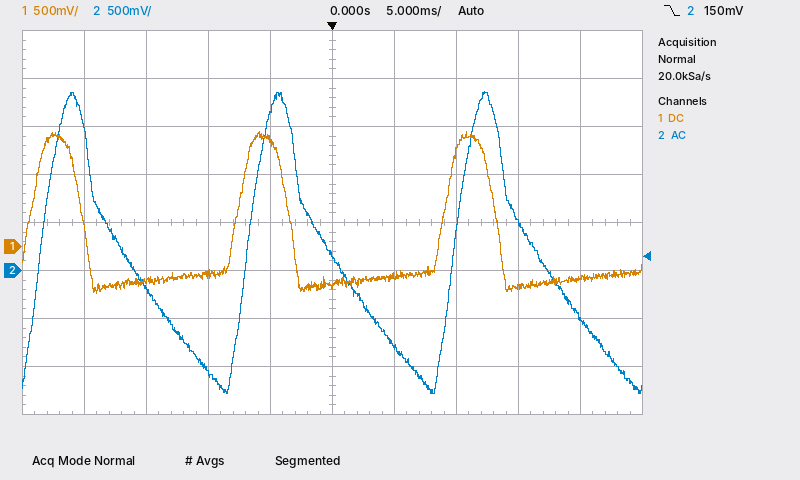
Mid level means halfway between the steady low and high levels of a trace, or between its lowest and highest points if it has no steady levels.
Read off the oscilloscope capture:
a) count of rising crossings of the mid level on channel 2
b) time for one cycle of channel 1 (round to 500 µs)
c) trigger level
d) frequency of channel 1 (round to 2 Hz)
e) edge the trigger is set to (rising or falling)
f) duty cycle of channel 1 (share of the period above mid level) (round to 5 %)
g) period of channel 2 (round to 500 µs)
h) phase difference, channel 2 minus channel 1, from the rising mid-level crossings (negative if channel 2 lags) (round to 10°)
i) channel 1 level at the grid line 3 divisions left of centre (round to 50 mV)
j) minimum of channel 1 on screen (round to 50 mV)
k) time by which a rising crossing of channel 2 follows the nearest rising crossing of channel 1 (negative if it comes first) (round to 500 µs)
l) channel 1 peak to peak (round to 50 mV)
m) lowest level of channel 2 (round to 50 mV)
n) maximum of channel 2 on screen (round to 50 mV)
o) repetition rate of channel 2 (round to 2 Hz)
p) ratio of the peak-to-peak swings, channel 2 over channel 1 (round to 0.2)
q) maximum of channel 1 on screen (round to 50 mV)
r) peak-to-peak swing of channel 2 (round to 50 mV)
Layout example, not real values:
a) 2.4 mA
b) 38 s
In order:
a) 3
b) 16.5 ms
c) 150 mV
d) 60 Hz
e) falling
f) 25 %
g) 16.5 ms
h) -20°
i) -350 mV
j) -500 mV
k) +1.0 ms
l) 1.70 V
m) -1.30 V
n) 1.85 V
o) 60 Hz
p) 1.8
q) 1.20 V
r) 3.15 V
